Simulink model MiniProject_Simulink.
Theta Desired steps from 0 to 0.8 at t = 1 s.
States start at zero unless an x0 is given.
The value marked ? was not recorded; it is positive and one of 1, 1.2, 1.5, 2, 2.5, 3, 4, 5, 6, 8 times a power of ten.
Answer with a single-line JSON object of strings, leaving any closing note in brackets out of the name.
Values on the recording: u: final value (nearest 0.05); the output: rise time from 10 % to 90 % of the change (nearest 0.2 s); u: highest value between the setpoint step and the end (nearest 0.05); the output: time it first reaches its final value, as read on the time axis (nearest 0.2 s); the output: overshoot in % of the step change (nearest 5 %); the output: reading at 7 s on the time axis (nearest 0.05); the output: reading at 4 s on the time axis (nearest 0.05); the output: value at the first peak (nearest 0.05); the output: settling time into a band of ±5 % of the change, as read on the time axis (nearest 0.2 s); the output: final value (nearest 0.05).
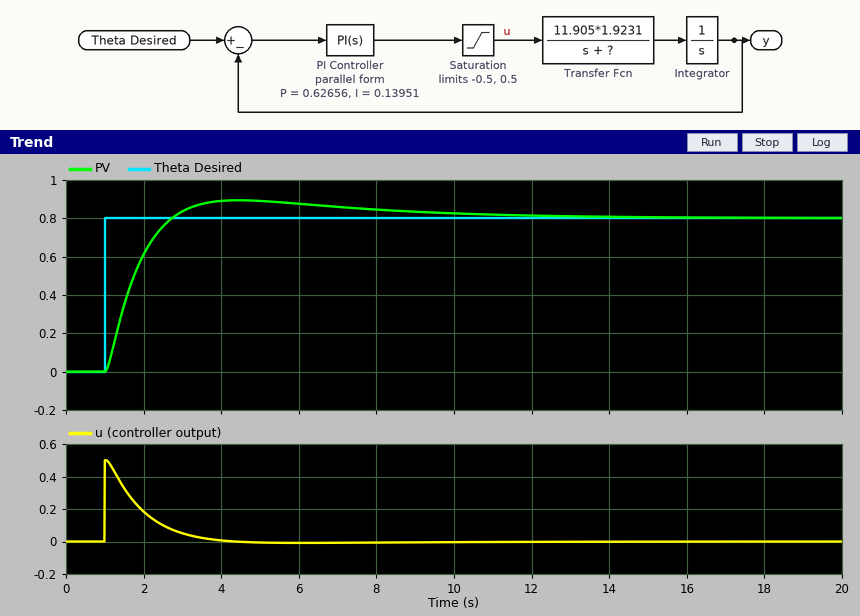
{"u: final value": "0.00", "the output: rise time from 10 % to 90 % of the change": "1.2 s", "u: highest value between the setpoint step and the end": "0.50", "the output: time it first reaches its final value, as read on the time axis": "2.8 s", "the output: overshoot in % of the step change": "10 %", "the output: reading at 7 s on the time axis": "0.85", "the output: reading at 4 s on the time axis": "0.90", "the output: value at the first peak": "0.90", "the output: settling time into a band of ±5 % of the change, as read on the time axis": "8.4 s", "the output: final value": "0.80"}
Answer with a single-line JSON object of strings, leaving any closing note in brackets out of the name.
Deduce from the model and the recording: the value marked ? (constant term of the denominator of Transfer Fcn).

{"the value marked ?": "12"}
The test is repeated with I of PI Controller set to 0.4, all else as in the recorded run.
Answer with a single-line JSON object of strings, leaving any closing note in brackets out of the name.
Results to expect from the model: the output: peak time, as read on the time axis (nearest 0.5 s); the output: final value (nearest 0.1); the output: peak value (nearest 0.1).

{"the output: peak time, as read on the time axis": "3.5 s", "the output: final value": "0.8", "the output: peak value": "1.0"}
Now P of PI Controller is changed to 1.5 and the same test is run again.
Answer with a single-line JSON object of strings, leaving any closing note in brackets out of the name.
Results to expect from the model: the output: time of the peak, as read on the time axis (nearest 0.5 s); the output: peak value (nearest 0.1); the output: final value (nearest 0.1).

{"the output: time of the peak, as read on the time axis": "3.0 s", "the output: peak value": "0.8", "the output: final value": "0.8"}
